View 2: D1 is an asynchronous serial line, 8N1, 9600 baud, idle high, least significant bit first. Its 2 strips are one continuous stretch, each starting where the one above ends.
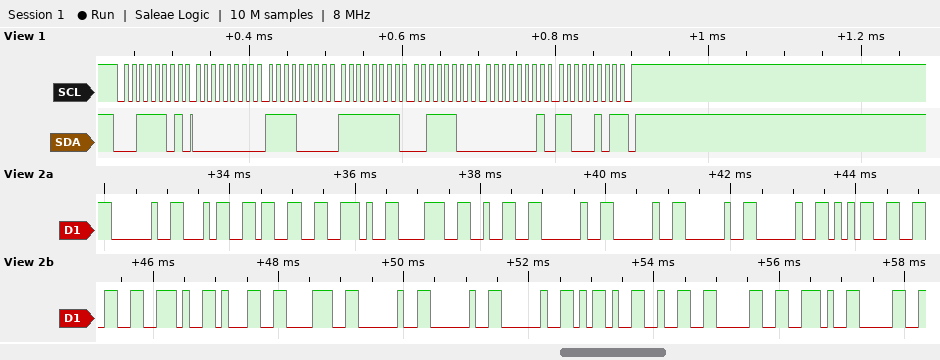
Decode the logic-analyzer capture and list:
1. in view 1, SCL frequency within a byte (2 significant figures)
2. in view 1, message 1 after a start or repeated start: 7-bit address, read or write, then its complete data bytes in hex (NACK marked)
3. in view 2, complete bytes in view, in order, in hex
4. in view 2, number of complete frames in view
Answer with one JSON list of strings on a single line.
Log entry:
["100 kHz", "0x1E read: 00 F0 FF 3C 01 C5 NACK", "20 34 33 2E 38 32 20 20 20 20 35 36 2E 31 38 20 20 20 2D 32 30 2E 30", "23"]
